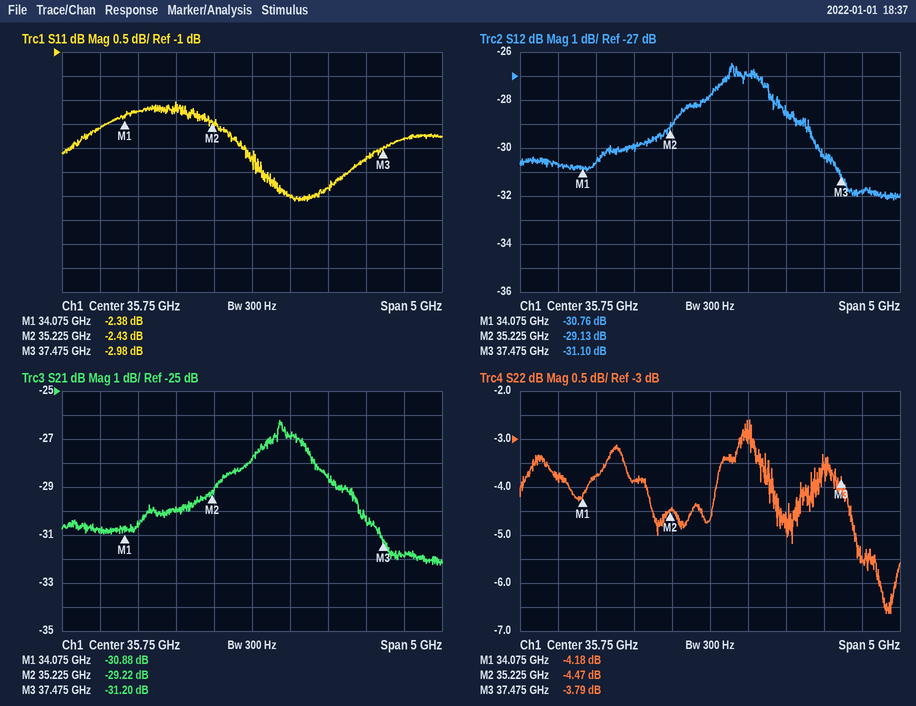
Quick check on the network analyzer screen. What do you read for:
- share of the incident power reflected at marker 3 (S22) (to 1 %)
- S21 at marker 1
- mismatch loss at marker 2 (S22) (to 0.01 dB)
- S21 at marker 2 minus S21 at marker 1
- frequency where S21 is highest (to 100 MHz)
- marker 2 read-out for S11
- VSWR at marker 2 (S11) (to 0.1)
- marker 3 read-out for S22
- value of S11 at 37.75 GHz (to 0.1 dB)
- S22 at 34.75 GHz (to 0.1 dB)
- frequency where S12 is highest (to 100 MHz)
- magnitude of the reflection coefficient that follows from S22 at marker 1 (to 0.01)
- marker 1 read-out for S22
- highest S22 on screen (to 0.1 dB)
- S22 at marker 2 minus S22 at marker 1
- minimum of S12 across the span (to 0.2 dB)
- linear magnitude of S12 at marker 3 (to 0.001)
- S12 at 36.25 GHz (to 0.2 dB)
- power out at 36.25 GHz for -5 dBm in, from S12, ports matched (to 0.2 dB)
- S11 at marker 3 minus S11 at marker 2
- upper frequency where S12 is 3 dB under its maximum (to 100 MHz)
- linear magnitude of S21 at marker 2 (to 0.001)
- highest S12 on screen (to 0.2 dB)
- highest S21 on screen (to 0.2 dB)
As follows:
42 %
-30.88 dB
1.92 dB
1.66 dB
36.1 GHz
-2.43 dB
7.2
-3.79 dB
-2.8 dB
-3.9 dB
36.0 GHz
0.62
-4.18 dB
-2.6 dB
-0.29 dB
-32.2 dB
0.028
-27.0 dB
-32.0 dBm
-0.55 dB
37.1 GHz
0.035
-26.4 dB
-26.2 dB
